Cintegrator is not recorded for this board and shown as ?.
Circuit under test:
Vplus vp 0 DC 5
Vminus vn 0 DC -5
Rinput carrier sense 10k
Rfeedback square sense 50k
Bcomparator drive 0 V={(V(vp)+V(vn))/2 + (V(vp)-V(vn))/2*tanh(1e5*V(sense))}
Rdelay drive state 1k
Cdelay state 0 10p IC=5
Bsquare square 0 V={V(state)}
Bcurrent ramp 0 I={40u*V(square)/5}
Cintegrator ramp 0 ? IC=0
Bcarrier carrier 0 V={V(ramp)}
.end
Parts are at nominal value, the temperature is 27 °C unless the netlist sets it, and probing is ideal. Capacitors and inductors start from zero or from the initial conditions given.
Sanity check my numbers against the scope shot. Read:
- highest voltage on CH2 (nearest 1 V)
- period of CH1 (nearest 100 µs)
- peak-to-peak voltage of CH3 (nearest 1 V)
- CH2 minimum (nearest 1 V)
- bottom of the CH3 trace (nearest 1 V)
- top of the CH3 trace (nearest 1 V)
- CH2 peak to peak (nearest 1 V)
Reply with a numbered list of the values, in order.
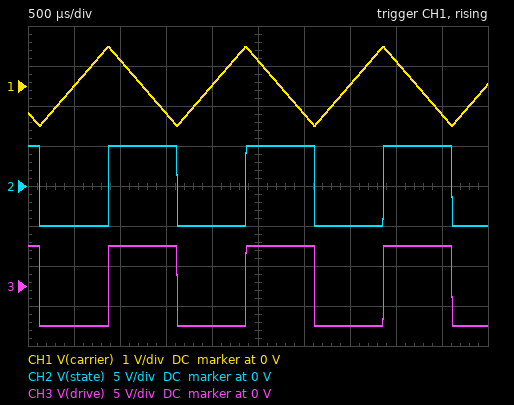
1. 5 V
2. 1.5 ms
3. 10 V
4. -5 V
5. -5 V
6. 5 V
7. 10 V
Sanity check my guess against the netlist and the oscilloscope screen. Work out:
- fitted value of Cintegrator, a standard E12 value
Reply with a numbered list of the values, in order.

1. 15 nF
